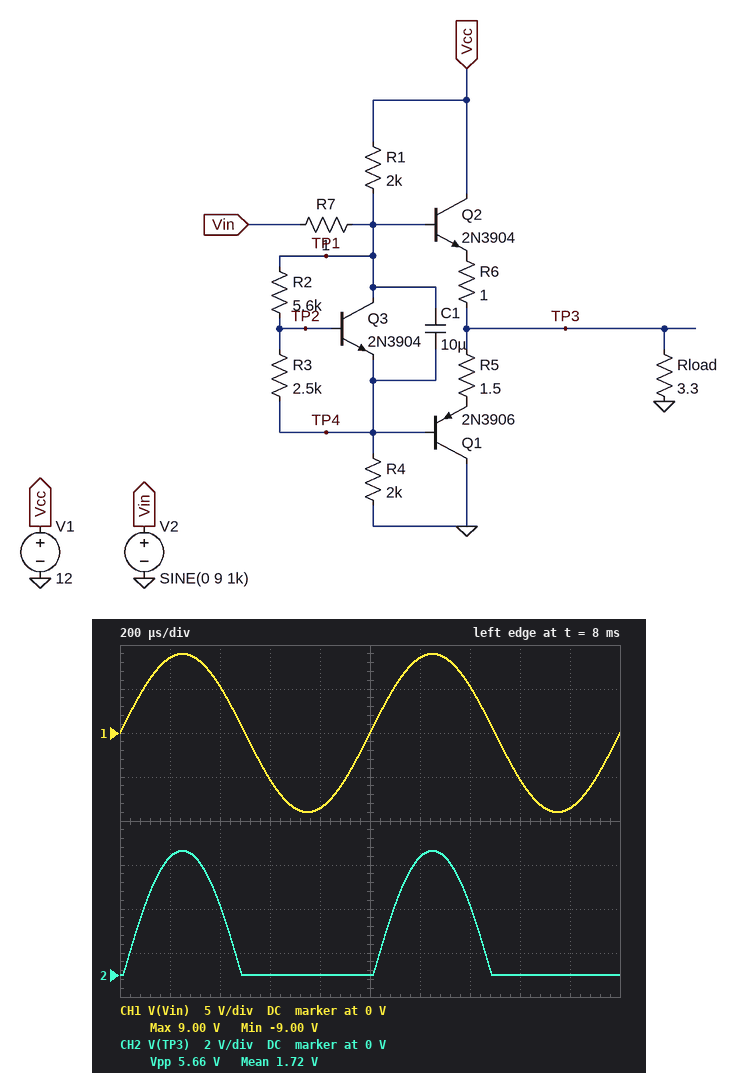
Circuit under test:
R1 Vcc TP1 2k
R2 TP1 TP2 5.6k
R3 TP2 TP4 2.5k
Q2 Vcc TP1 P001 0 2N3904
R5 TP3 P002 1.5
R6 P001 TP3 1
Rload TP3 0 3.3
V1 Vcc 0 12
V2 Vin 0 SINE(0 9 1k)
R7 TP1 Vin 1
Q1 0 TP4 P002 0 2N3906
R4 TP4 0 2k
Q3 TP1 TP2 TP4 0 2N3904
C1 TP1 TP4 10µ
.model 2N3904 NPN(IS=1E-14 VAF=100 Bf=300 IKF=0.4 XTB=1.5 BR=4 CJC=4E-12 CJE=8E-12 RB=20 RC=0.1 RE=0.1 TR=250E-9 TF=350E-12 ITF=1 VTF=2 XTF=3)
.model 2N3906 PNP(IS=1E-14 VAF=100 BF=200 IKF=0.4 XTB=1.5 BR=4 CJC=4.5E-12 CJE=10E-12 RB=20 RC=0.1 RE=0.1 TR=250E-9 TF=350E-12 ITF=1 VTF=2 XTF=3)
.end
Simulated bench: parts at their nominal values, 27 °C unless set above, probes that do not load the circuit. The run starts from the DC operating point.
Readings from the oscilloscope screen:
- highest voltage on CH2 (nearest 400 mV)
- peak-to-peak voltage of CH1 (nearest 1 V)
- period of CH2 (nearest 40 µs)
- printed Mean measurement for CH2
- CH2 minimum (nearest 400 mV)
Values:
5.6 V
18 V
1.00 ms
1.72 V
0 V
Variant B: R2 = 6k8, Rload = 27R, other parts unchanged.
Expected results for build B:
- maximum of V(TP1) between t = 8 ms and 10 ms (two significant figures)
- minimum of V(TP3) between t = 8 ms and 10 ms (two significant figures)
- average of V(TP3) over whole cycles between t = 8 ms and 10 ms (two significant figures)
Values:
9.0 V
-8.9 mV
2.4 V
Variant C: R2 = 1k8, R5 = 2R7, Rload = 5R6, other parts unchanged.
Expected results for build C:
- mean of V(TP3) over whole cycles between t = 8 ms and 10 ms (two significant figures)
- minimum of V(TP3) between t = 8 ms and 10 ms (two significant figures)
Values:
2.0 V
-5.9 mV
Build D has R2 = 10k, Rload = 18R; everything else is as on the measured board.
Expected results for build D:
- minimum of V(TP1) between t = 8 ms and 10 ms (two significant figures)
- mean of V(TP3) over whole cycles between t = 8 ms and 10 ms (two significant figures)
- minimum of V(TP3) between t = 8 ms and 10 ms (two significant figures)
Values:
-8.9 V
2.3 V
-8.6 mV
